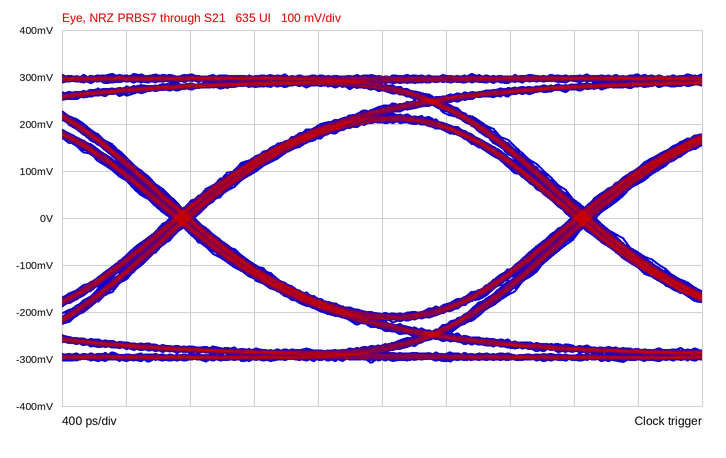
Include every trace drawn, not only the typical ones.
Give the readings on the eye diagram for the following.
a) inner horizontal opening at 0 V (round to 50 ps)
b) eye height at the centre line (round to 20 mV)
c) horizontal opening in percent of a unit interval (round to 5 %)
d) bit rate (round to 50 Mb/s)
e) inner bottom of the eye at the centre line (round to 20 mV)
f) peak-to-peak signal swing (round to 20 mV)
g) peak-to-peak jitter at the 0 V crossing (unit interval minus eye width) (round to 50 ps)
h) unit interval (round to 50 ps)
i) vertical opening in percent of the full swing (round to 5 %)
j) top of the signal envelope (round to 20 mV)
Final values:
2.35 ns
400 mV
95 %
400 Mb/s
-200 mV
620 mV
150 ps
2.50 ns
65 %
300 mV
